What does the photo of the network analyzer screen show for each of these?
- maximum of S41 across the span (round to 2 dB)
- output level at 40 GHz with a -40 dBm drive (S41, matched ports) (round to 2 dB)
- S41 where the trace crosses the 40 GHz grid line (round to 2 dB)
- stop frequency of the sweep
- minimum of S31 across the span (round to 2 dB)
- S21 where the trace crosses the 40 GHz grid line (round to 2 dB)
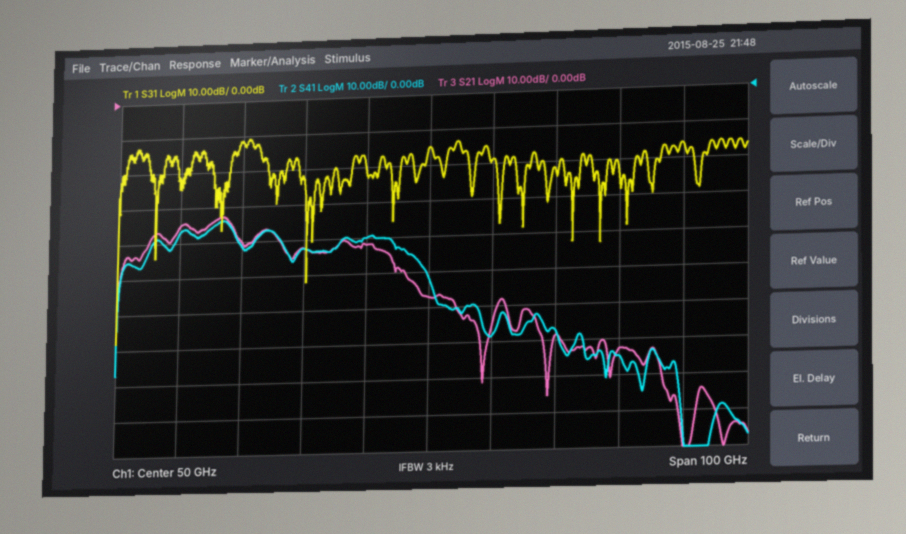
-34 dB
-80 dBm
-40 dB
100 GHz
-68 dB
-42 dB
